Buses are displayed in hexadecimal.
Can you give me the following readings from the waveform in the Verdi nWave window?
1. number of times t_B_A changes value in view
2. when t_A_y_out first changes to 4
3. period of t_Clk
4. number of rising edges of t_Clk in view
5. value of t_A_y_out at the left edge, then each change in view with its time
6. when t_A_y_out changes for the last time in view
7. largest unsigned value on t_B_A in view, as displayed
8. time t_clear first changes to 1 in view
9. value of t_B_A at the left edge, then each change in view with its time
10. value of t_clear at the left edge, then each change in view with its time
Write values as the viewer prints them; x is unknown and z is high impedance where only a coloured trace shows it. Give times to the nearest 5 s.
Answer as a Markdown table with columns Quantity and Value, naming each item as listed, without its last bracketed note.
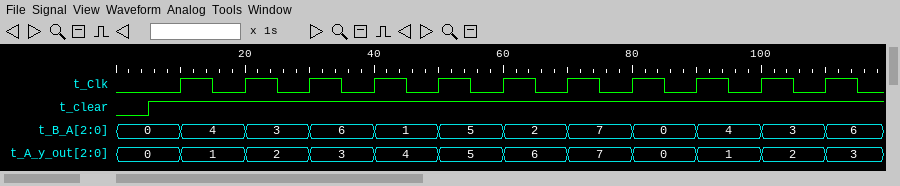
| Quantity | Value |
|---|---|
| number of times t_B_A changes value in view | 11 |
| when t_A_y_out first changes to 4 | 40 s |
| period of t_Clk | 10 s |
| number of rising edges of t_Clk in view | 11 |
| value of t_A_y_out at the left edge, then each change in view with its time | 0, 1 at 10 s, 2 at 20 s, 3 at 30 s, 4 at 40 s, 5 at 50 s, 6 at 60 s, 7 at 70 s, 0 at 80 s, 1 at 90 s, 2 at 100 s, 3 at 110 s |
| when t_A_y_out changes for the last time in view | 110 s |
| largest unsigned value on t_B_A in view, as displayed | 7 |
| time t_clear first changes to 1 in view | 5 s |
| value of t_B_A at the left edge, then each change in view with its time | 0, 4 at 10 s, 3 at 20 s, 6 at 30 s, 1 at 40 s, 5 at 50 s, 2 at 60 s, 7 at 70 s, 0 at 80 s, 4 at 90 s, 3 at 100 s, 6 at 110 s |
| value of t_clear at the left edge, then each change in view with its time | 0, 1 at 5 s |
